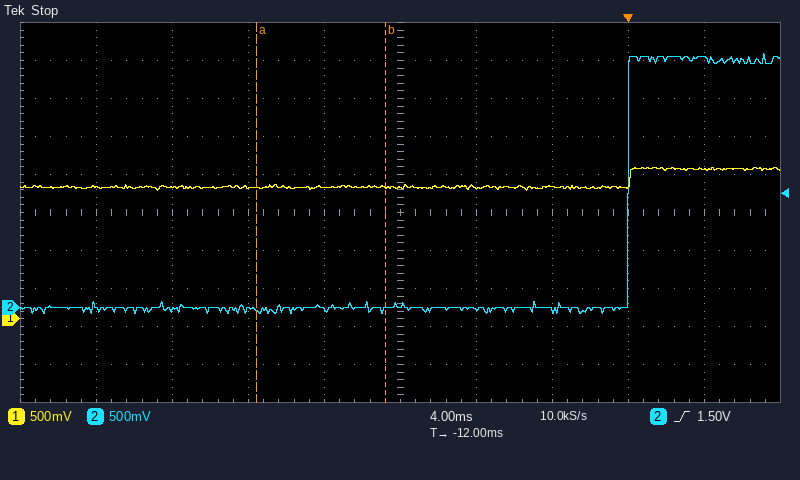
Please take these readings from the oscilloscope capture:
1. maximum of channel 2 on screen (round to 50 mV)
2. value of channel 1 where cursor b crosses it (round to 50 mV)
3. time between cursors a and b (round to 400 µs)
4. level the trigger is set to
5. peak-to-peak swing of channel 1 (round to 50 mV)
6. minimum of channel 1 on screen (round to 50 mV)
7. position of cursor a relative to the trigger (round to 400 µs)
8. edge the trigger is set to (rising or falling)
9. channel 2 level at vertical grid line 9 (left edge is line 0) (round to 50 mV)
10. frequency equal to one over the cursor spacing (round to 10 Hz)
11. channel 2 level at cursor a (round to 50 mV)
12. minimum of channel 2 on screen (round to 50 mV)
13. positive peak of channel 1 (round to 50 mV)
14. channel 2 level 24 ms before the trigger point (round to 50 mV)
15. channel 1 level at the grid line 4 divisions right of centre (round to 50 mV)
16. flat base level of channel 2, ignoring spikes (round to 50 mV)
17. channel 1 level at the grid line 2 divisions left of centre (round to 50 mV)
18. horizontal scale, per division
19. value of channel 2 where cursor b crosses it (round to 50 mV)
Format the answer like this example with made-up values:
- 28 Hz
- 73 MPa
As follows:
- 3.35 V
- 1.75 V
- 6.8 ms
- 1.50 V
- 300 mV
- 1.70 V
- -19.6 ms
- rising
- 3.25 V
- 150 Hz
- -50 mV
- -100 mV
- 2.00 V
- -50 mV
- 1.95 V
- 0 mV
- 1.75 V
- 4 ms
- -50 mV
